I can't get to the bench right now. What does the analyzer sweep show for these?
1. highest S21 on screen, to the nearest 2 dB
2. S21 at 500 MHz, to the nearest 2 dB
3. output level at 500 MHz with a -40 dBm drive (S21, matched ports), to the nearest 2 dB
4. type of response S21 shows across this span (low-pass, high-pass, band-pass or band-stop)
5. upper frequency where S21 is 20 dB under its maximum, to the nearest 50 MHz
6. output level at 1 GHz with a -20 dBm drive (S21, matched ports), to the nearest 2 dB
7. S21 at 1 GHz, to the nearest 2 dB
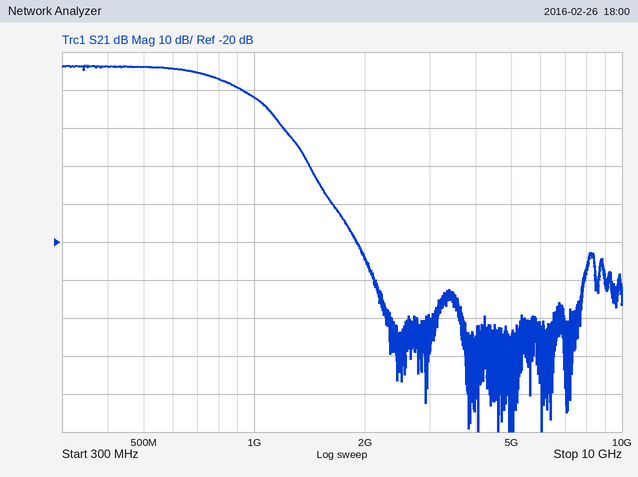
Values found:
26 dB
26 dB
-14 dBm
low-pass
1.30 GHz
-2 dBm
18 dB
